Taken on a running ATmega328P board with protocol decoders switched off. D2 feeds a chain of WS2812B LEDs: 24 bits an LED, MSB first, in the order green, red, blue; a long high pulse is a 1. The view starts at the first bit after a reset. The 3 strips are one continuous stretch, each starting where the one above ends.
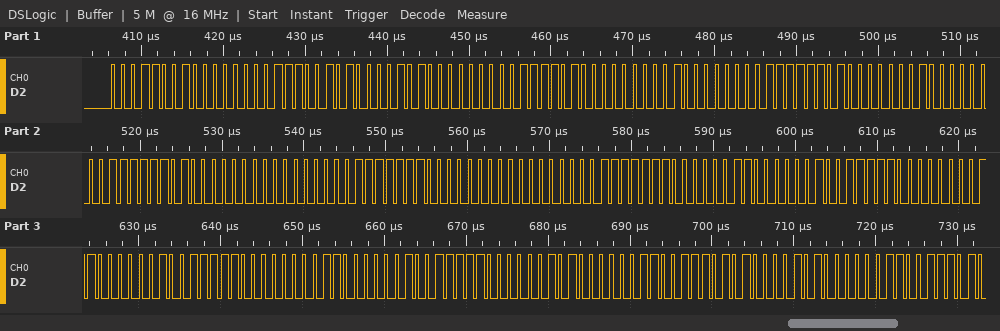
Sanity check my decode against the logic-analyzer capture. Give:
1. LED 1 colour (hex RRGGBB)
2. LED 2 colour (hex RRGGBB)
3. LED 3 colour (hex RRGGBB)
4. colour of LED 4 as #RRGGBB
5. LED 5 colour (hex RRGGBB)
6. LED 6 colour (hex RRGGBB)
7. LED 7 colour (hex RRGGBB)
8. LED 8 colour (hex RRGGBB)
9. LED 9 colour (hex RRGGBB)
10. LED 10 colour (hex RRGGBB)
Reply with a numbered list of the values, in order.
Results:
1. #0019E5
2. #000AF4
3. #0001FD
4. #0001FD
5. #0000FE
6. #0000FE
7. #0406F8
8. #0406F8
9. #0406F8
10. #0C14EA
